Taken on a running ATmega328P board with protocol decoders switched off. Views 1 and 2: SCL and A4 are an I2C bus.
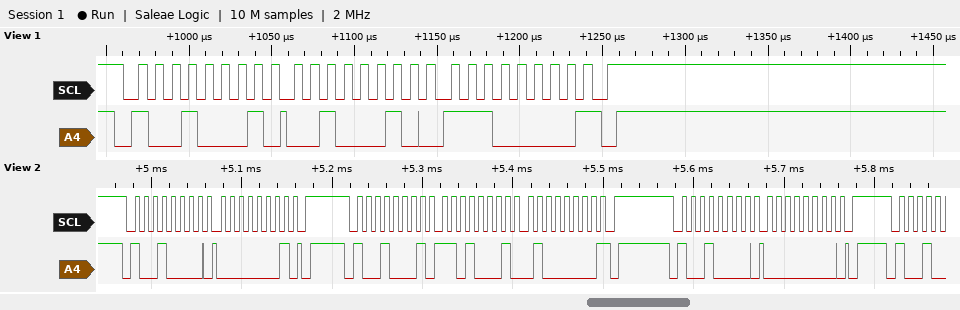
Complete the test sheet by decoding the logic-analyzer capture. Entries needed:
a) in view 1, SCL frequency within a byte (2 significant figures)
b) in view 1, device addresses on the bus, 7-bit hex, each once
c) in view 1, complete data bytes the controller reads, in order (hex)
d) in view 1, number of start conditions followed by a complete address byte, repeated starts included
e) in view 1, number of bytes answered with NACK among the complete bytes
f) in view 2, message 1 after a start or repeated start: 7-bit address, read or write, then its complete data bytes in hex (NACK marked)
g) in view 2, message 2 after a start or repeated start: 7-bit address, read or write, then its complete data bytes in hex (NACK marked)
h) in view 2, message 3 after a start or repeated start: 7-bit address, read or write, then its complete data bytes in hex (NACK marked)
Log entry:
100 kHz
0x48
22 E0
1
1
0x48 write: 01
0x48 read: D1 40 NACK
0x48 write: 00
